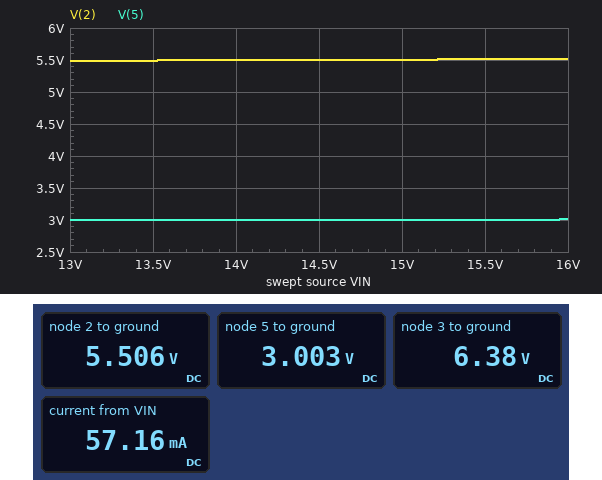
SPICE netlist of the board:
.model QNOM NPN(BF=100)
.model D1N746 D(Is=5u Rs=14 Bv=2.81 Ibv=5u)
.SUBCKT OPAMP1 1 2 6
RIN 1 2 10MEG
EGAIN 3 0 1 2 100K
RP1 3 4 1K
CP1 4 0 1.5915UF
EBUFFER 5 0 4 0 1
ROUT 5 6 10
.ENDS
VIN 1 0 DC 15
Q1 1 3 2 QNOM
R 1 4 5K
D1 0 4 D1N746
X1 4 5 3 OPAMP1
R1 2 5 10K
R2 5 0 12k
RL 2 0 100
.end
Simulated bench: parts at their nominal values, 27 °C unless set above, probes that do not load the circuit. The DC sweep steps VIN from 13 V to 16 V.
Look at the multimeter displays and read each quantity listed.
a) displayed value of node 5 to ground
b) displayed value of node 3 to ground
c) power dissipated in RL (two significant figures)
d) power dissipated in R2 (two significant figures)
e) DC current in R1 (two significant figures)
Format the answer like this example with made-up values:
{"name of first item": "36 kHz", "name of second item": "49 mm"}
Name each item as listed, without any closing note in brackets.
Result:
{"displayed value of node 5 to ground": "3.003 V", "displayed value of node 3 to ground": "6.38 V", "power dissipated in RL": "300 mW", "power dissipated in R2": "750 µW", "DC current in R1": "250 µA"}
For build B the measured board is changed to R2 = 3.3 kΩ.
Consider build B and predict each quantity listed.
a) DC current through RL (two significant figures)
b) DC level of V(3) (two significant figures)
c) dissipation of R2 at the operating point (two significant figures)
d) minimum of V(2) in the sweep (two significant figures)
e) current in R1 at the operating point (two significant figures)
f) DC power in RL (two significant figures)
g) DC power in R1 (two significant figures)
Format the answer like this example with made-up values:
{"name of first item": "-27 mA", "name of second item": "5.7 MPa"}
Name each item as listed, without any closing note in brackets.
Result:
{"DC current through RL": "120 mA", "DC level of V(3)": "13 V", "dissipation of R2 at the operating point": "2.7 mW", "minimum of V(2) in the sweep": "12 V", "current in R1 at the operating point": "910 µA", "DC power in RL": "1.5 W", "DC power in R1": "8.3 mW"}
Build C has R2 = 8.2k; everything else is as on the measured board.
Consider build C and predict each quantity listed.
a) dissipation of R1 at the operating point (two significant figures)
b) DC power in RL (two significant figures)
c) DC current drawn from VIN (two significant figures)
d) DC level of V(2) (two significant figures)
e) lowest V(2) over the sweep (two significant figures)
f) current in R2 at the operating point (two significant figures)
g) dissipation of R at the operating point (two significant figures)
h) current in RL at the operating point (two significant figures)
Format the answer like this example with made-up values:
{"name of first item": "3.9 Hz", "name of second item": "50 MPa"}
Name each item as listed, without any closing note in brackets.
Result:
{"dissipation of R1 at the operating point": "1.3 mW", "DC power in RL": "440 mW", "DC current drawn from VIN": "69 mA", "DC level of V(2)": "6.7 V", "lowest V(2) over the sweep": "6.6 V", "current in R2 at the operating point": "370 µA", "dissipation of R at the operating point": "29 mW", "current in RL at the operating point": "67 mA"}
